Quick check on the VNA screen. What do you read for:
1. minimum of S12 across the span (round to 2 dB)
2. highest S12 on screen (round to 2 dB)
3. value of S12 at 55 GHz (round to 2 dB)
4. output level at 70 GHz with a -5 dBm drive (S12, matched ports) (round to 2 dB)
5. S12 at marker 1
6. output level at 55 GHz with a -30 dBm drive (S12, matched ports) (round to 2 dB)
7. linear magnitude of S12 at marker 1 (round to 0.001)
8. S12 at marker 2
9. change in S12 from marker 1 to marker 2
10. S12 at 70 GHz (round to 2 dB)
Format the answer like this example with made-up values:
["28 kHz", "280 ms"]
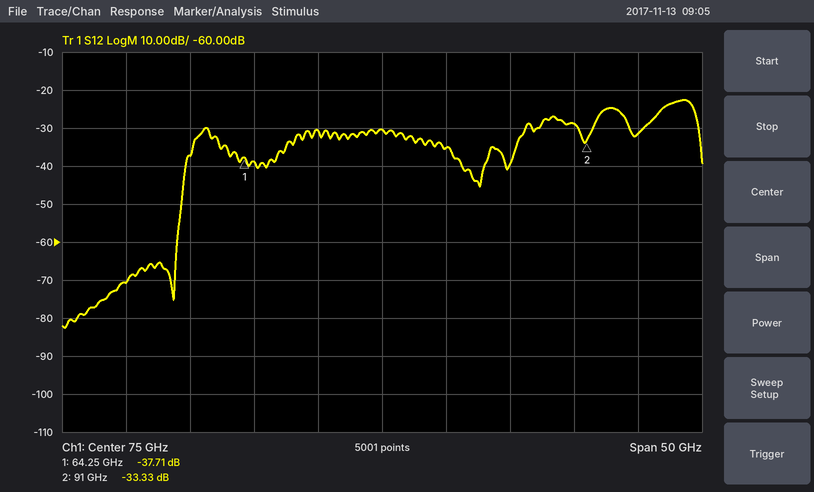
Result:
["-82 dB", "-22 dB", "-70 dB", "-36 dBm", "-37.71 dB", "-100 dBm", "0.013", "-33.33 dB", "4.38 dB", "-30 dB"]
